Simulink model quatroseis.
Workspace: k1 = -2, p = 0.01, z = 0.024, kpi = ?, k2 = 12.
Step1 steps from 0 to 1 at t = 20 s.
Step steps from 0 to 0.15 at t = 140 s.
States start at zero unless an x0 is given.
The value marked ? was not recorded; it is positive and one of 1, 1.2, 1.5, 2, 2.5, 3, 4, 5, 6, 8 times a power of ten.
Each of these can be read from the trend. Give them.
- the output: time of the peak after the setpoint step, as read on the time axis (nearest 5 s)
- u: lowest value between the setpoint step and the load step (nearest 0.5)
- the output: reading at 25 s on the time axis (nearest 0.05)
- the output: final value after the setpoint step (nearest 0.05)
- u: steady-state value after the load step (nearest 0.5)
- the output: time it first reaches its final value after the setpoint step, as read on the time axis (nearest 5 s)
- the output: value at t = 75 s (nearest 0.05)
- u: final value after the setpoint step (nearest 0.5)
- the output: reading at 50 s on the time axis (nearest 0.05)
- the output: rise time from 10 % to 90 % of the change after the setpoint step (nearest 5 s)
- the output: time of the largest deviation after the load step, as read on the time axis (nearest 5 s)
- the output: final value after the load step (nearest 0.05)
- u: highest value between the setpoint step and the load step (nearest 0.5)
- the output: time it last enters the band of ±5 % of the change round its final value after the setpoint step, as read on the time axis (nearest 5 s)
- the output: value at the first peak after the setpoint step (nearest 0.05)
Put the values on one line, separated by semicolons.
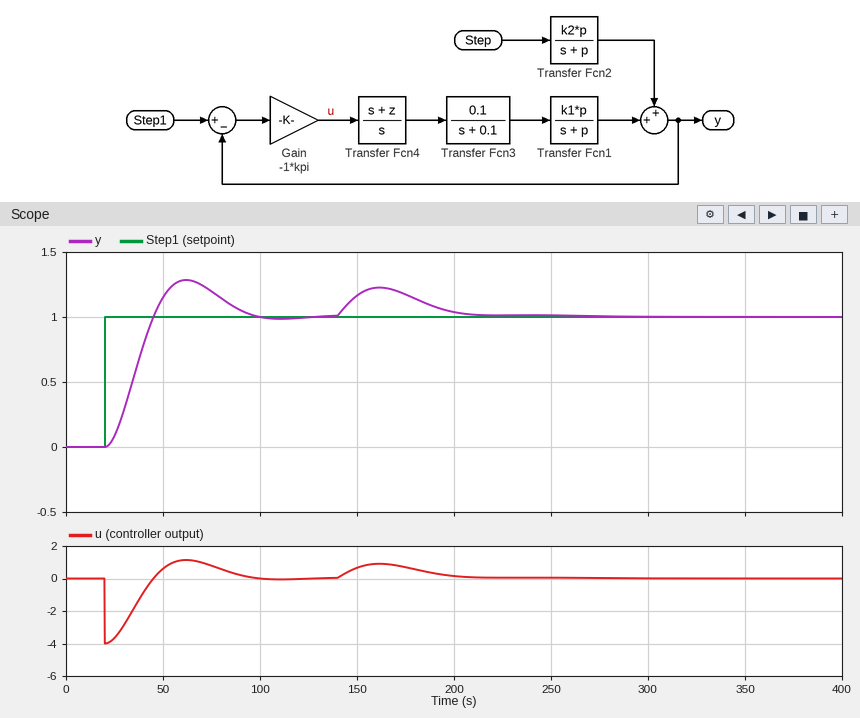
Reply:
60 s; -4.0; 0.10; 1.00; 0.0; 45 s; 1.20; 0.0; 1.15; 15 s; 160 s; 1.00; 1.0; 90 s; 1.30
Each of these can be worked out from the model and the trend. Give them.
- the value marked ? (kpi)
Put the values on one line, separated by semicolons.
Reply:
4
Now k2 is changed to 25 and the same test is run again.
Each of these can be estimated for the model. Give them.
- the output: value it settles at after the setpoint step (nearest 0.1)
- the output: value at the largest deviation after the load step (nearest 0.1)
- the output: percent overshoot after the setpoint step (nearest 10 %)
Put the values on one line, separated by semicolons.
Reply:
1.0; 1.5; 30 %
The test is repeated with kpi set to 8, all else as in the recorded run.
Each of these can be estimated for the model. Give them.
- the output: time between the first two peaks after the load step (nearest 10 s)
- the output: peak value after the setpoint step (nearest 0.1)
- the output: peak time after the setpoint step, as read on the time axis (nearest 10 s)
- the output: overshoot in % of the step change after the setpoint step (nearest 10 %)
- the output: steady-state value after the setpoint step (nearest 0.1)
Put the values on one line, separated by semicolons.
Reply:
50 s; 1.4; 50 s; 40 %; 1.0
